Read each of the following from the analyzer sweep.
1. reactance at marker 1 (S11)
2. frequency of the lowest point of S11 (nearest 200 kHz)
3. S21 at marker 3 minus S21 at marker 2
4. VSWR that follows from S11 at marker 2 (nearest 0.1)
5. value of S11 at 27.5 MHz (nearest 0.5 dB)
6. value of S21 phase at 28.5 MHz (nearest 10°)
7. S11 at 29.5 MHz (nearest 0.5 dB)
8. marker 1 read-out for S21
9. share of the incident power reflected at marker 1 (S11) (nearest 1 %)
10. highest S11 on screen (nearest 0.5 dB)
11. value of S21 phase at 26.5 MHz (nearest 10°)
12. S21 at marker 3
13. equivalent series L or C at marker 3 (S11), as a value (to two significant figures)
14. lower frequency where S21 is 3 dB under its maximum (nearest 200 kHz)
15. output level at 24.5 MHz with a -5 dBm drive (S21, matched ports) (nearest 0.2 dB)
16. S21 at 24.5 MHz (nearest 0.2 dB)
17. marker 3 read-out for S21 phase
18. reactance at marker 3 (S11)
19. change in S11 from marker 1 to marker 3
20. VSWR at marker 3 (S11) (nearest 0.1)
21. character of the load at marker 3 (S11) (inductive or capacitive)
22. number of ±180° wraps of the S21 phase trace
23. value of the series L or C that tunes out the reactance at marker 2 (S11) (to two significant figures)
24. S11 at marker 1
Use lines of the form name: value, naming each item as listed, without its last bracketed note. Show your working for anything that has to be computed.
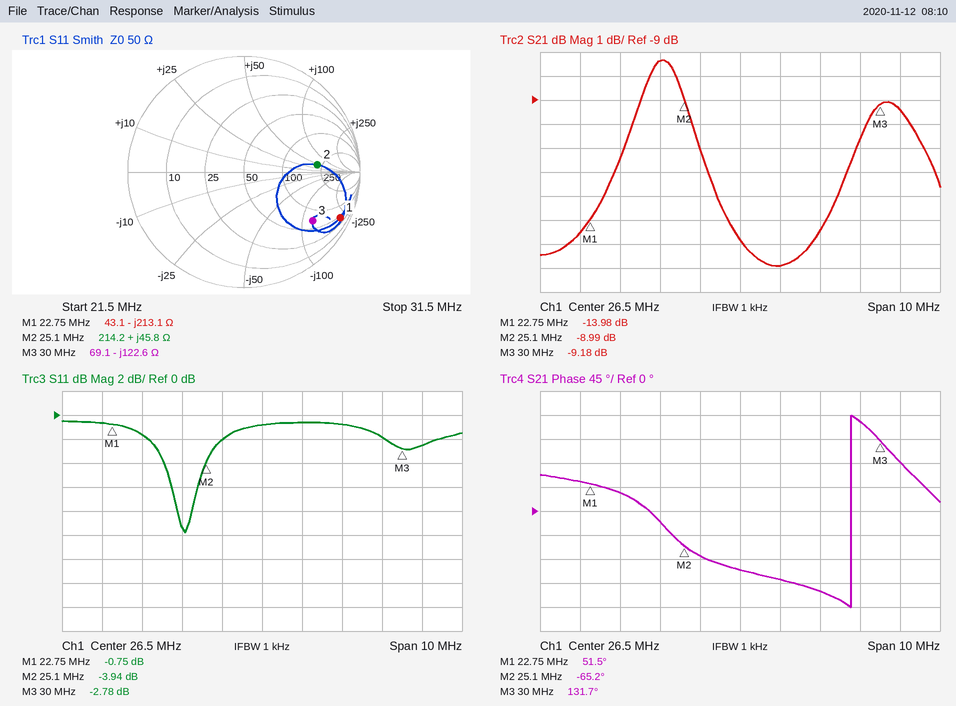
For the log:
reactance at marker 1: -213.1 Ω
frequency of the lowest point of S11: 24.6 MHz
S21 at marker 3 minus S21 at marker 2: -9.18 − (-8.99) = -0.19 dB
VSWR that follows from S11 at marker 2: (1 + 0.6353)/(1 − 0.6353) ≈ 4.5
value of S11 at 27.5 MHz: -0.5 dB
value of S21 phase at 28.5 MHz: -150°
S11 at 29.5 MHz: -2.0 dB
marker 1 read-out for S21: -13.98 dB
share of the incident power reflected at marker 1 (S11): 10^(-0.75/10) ≈ 84 %
highest S11 on screen: -0.5 dB
value of S21 phase at 26.5 MHz: -110°
S21 at marker 3: -9.18 dB
equivalent series L or C at marker 3 (S11), as a value: C = 1/(2π × 30 MHz × 122.6 Ω) ≈ 43 pF
lower frequency where S21 is 3 dB under its maximum: 23.8 MHz
output level at 24.5 MHz with a -5 dBm drive (S21, matched ports): -5 dBm + (-7.4 dB) = -12.4 dBm
S21 at 24.5 MHz: -7.4 dB
marker 3 read-out for S21 phase: 131.7°
reactance at marker 3: -122.6 Ω
change in S11 from marker 1 to marker 3: -2.78 − (-0.75) = -2.03 dB
VSWR at marker 3 (S11): 6.3
character of the load at marker 3 (S11): capacitive
number of ±180° wraps of the S21 phase trace: 1
value of the series L or C that tunes out the reactance at marker 2 (S11): C = 1/(2π × 25.1 MHz × 45.8 Ω) ≈ 138 pF, so 140 pF to two significant figures
S11 at marker 1: -0.75 dB
